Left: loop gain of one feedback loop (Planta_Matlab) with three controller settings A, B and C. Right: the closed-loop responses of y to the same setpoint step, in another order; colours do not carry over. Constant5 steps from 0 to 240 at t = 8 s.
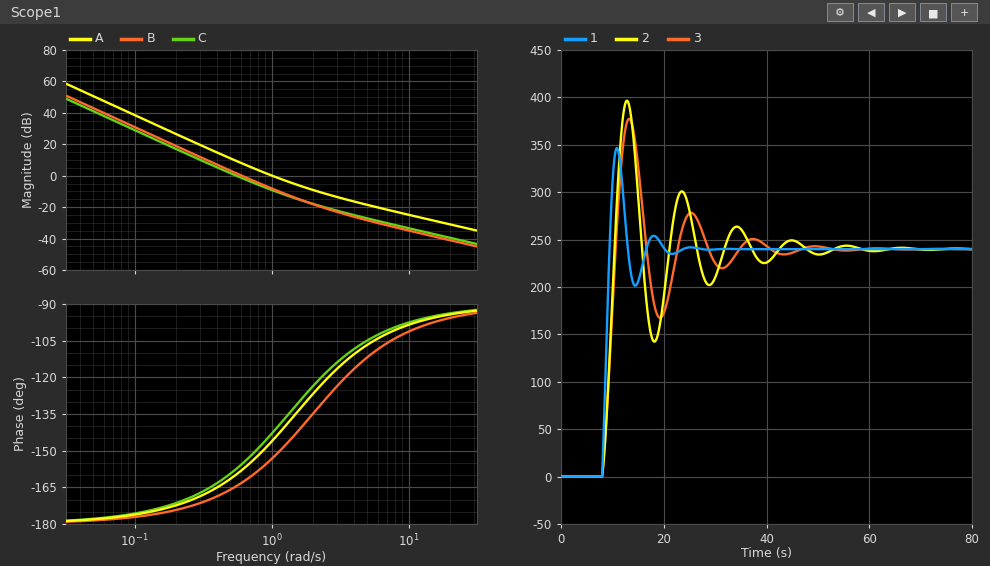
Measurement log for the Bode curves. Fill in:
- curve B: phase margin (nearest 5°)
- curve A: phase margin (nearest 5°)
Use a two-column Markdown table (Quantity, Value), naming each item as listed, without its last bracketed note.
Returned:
| Quantity | Value |
|---|---|
| curve B: phase margin | 15° |
| curve A: phase margin | 35° |
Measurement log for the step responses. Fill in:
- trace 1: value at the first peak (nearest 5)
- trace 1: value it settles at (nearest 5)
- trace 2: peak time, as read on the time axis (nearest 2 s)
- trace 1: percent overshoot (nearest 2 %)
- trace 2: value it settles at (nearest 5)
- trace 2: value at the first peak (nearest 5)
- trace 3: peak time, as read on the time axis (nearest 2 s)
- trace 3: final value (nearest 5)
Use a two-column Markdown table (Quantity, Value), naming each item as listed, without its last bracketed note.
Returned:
| Quantity | Value |
|---|---|
| trace 1: value at the first peak | 345 |
| trace 1: value it settles at | 240 |
| trace 2: peak time, as read on the time axis | 12 s |
| trace 1: percent overshoot | 44 % |
| trace 2: value it settles at | 240 |
| trace 2: value at the first peak | 395 |
| trace 3: peak time, as read on the time axis | 14 s |
| trace 3: final value | 240 |
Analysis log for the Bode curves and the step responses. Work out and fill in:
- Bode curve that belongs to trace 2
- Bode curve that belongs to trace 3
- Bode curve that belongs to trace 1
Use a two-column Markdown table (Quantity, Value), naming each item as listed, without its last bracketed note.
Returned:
| Quantity | Value |
|---|---|
| Bode curve that belongs to trace 2 | B |
| Bode curve that belongs to trace 3 | C |
| Bode curve that belongs to trace 1 | A |
